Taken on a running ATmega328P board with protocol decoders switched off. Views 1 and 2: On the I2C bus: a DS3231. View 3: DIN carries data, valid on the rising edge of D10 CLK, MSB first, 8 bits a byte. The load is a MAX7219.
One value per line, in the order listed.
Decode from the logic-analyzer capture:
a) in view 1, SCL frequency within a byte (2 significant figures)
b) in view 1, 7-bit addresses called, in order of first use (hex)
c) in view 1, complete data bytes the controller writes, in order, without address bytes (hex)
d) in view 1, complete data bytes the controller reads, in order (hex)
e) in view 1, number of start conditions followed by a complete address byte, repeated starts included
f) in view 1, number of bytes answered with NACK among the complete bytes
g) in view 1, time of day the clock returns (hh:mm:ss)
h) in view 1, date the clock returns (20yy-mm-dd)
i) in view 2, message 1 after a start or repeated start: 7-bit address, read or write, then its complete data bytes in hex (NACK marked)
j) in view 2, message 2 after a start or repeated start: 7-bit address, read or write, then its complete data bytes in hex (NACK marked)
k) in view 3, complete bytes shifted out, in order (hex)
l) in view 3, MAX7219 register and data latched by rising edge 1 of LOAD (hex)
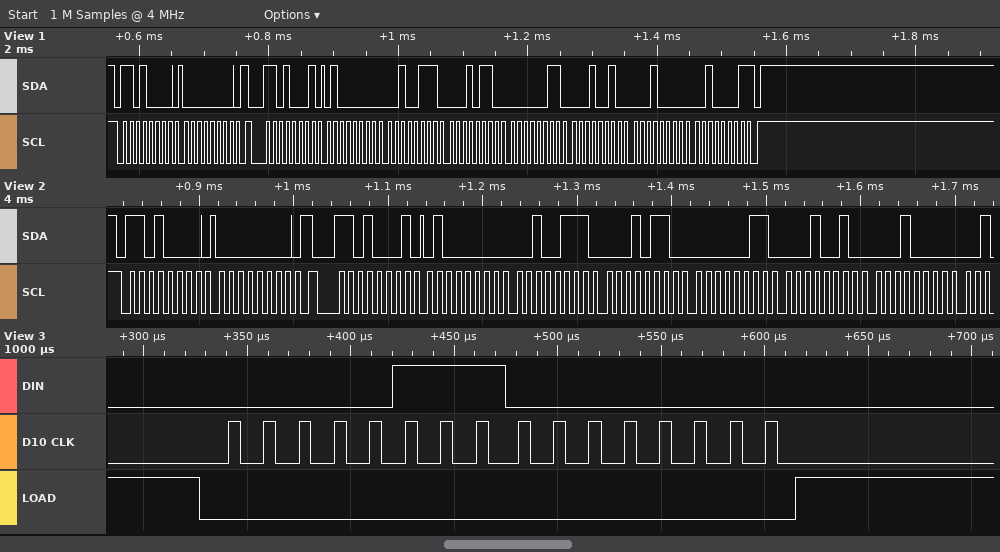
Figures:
100 kHz
0x68
00
40 27 16 03 12 10 21
2
1
16:27:40
2021-10-12
0x68 write: 00
0x68 read: 40 27 16 03 12 10
0x07 0x00
register 0x7, data 0x00
